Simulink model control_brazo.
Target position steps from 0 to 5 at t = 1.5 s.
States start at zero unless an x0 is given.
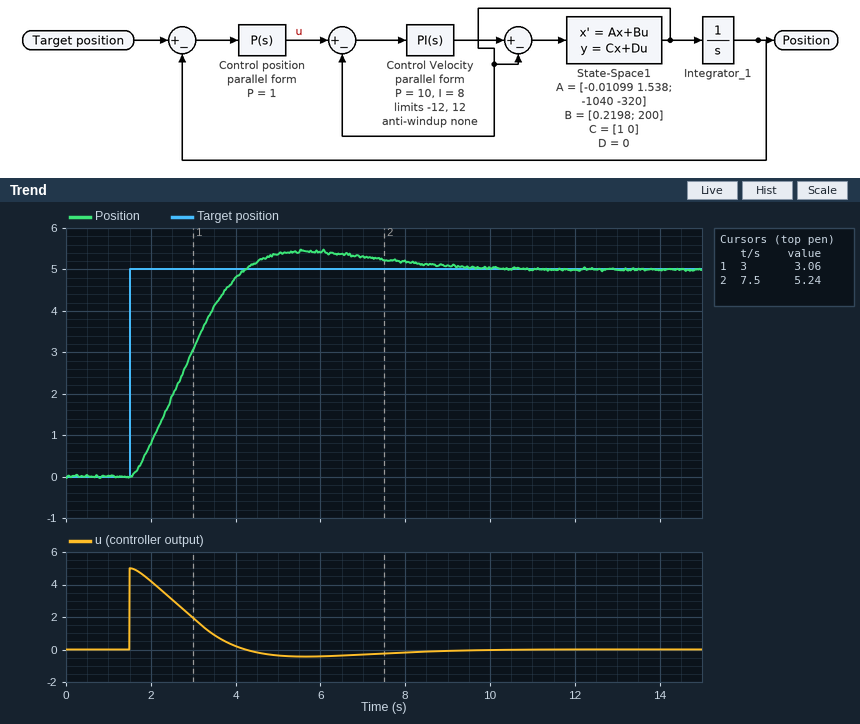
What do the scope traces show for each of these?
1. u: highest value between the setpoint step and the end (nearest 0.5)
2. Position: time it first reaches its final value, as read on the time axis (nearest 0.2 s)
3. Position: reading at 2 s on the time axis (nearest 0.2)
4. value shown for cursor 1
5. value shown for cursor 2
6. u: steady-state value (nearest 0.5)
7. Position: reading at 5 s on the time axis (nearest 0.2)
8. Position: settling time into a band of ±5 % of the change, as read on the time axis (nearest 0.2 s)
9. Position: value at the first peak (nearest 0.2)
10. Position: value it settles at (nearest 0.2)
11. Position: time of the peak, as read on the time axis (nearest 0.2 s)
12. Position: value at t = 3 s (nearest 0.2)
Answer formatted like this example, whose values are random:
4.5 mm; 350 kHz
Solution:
5.0; 4.2 s; 0.8; 3.06; 5.24; 0.0; 5.4; 7.4 s; 5.4; 5.0; 5.6 s; 3.0
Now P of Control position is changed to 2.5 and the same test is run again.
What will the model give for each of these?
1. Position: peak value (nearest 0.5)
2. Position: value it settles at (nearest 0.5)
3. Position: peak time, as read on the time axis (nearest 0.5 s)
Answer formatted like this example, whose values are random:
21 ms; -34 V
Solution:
7.0; 5.0; 5.0 s
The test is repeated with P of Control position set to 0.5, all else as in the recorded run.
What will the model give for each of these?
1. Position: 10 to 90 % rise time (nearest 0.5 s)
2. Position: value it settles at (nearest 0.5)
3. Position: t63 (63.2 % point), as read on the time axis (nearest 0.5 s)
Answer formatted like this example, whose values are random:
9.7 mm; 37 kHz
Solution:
4.0 s; 5.0; 4.0 s
